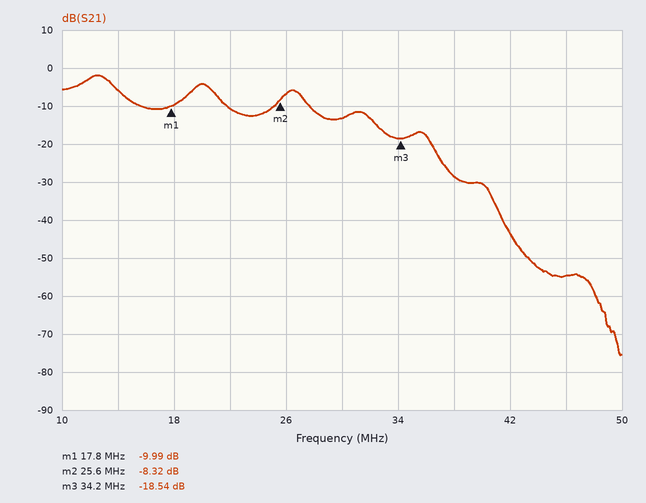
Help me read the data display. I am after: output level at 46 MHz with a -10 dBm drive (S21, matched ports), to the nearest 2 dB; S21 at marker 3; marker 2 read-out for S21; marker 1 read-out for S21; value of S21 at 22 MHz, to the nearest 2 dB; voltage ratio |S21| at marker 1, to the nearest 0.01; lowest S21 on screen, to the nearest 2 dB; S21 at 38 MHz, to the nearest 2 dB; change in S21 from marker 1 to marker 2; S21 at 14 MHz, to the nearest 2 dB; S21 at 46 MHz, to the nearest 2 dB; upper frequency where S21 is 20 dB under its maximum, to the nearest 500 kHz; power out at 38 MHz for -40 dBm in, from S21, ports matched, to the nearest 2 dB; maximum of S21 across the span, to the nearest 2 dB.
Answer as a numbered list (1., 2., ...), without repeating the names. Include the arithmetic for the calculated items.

1. -10 dBm + (-54 dB) = -64 dBm
2. -18.54 dB
3. -8.32 dB
4. -9.99 dB
5. -10 dB
6. 10^(-9.99/20) ≈ 0.32
7. -76 dB
8. -28 dB
9. -8.32 − (-9.99) = 1.67 dB
10. -6 dB
11. -54 dB
12. 36.5 MHz
13. -40 dBm + (-28 dB) = -68 dBm
14. -2 dB
